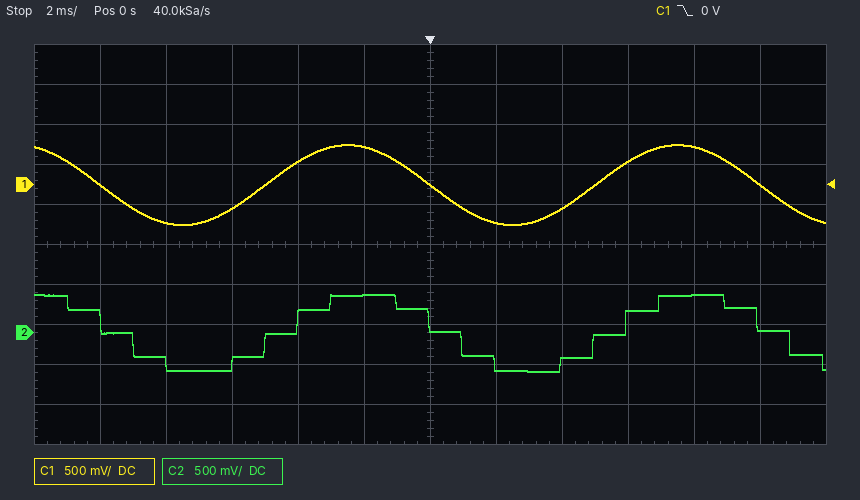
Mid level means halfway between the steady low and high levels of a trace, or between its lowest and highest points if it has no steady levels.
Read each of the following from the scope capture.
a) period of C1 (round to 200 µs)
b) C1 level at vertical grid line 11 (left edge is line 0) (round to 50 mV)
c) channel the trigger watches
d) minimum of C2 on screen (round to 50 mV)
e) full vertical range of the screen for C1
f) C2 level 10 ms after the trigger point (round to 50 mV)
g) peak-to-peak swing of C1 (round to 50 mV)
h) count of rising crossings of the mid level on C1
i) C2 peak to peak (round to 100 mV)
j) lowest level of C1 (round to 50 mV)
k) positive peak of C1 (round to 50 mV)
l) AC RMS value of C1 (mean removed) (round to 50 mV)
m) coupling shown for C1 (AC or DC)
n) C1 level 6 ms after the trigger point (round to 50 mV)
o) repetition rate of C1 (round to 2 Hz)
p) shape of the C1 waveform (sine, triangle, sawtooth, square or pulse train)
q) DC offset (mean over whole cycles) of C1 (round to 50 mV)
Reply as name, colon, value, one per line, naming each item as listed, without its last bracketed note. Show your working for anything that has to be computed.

period of C1: 10.0 ms
C1 level at vertical grid line 11 (left edge is line 0): 0 mV
channel the trigger watches: C1
minimum of C2 on screen: -500 mV
full vertical range of the screen for C1: 5 V
C2 level 10 ms after the trigger point: 50 mV
peak-to-peak swing of C1: 500 mV − (-500 mV) = 1.00 V
count of rising crossings of the mid level on C1: 2
C2 peak to peak: 1.00 V
lowest level of C1: -500 mV
positive peak of C1: 500 mV
AC RMS value of C1 (mean removed): 1.00 V / (2√2) ≈ 354 mV, so 350 mV to the nearest 50 mV
coupling shown for C1: DC
C1 level 6 ms after the trigger point: 300 mV
repetition rate of C1: 1 / 10.0 ms ≈ 100 Hz
shape of the C1 waveform: sine
DC offset (mean over whole cycles) of C1: (500 mV + (-500 mV)) / 2 ≈ 0 mV
